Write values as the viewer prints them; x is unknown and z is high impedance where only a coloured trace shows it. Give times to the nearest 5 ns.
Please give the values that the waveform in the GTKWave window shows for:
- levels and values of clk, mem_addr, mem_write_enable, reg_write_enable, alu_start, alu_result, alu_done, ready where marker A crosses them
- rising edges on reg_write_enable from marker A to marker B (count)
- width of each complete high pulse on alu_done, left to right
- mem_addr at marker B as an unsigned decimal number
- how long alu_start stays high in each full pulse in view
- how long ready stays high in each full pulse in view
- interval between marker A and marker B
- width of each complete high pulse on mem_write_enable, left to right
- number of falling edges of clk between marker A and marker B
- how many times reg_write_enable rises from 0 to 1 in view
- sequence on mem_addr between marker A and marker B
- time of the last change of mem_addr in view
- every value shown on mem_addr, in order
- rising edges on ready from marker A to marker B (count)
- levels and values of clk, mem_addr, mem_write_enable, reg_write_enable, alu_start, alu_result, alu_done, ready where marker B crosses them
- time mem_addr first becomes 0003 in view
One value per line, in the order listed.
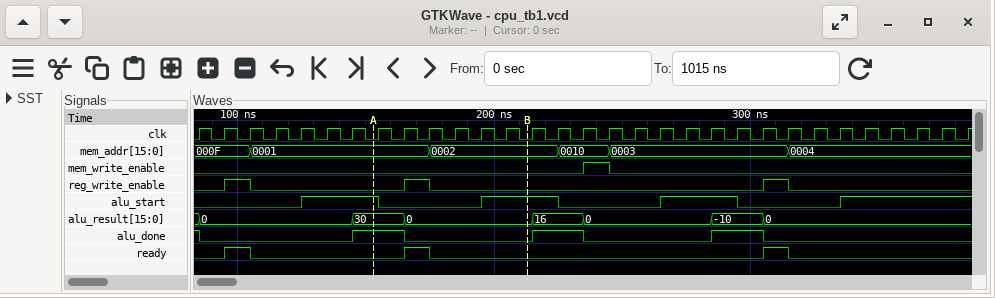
clk=0, mem_addr=0001, mem_write_enable=0, reg_write_enable=0, alu_start=1, alu_result=30, alu_done=1, ready=0
1
20 ns, 20 ns, 20 ns
2
30 ns, 30 ns, 30 ns
10 ns, 10 ns, 10 ns
60 ns
10 ns
6
3
0001, 0002
315 ns
000F, 0001, 0002, 0010, 0003, 0004
1
clk=0, mem_addr=0002, mem_write_enable=0, reg_write_enable=0, alu_start=1, alu_result=0, alu_done=0, ready=0
245 ns
